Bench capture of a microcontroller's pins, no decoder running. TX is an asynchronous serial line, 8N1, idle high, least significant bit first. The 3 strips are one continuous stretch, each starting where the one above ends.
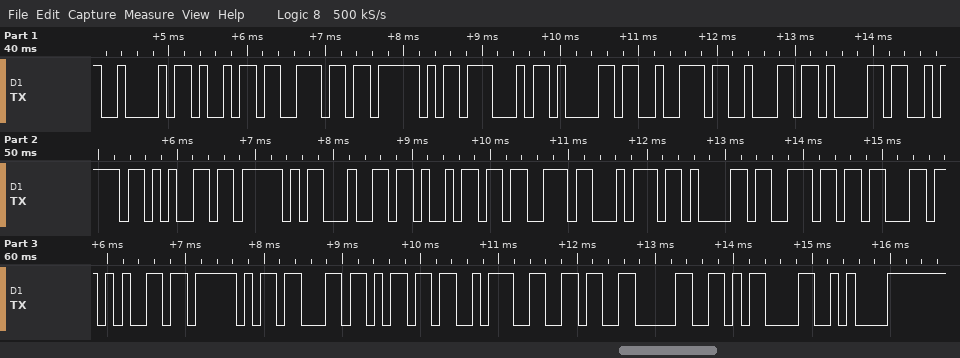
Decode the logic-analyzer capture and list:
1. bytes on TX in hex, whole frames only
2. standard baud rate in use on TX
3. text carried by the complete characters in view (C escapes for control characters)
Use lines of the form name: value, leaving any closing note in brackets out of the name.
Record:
bytes on TX in hex, whole frames only: 0x42 0x69 0x6E 0x5F 0x47 0x61 0x72 0x62 0x61 0x7A 0x65 0x5F 0x64 0x69 0x73 0x74 0x61 0x6E 0x63 0x65 0x5F 0x63 0x6D 0x3A 0x36 0x30 0x0D 0x0A
standard baud rate in use on TX: 9600 baud
text carried by the complete characters in view: "Bin_Garbaze_distance_cm:60\r\n"
